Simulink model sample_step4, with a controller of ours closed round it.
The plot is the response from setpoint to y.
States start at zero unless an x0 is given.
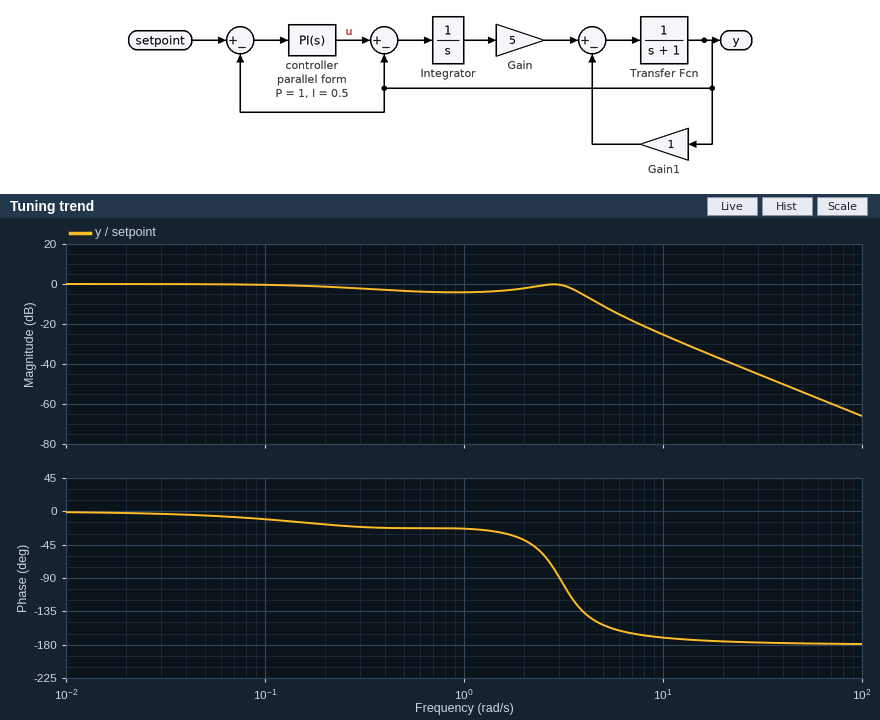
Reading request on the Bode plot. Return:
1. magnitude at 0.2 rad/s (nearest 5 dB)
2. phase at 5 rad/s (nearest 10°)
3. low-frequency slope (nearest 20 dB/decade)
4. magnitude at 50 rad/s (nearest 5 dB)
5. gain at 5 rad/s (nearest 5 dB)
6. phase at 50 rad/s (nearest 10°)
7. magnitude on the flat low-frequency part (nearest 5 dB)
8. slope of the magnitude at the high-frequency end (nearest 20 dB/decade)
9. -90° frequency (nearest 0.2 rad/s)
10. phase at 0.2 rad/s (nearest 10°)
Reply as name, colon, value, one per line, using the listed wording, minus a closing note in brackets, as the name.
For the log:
magnitude at 0.2 rad/s: 0 dB
phase at 5 rad/s: -150°
low-frequency slope: 0 dB/decade
magnitude at 50 rad/s: -55 dB
gain at 5 rad/s: -10 dB
phase at 50 rad/s: -180°
magnitude on the flat low-frequency part: 0 dB
slope of the magnitude at the high-frequency end: -40 dB/decade
-90° frequency: 3.0 rad/s
phase at 0.2 rad/s: -20°
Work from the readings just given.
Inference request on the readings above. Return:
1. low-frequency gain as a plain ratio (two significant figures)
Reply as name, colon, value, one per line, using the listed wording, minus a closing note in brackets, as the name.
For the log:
low-frequency gain as a plain ratio: 1.0
